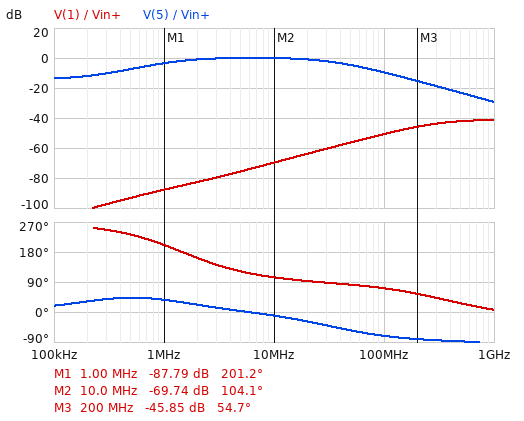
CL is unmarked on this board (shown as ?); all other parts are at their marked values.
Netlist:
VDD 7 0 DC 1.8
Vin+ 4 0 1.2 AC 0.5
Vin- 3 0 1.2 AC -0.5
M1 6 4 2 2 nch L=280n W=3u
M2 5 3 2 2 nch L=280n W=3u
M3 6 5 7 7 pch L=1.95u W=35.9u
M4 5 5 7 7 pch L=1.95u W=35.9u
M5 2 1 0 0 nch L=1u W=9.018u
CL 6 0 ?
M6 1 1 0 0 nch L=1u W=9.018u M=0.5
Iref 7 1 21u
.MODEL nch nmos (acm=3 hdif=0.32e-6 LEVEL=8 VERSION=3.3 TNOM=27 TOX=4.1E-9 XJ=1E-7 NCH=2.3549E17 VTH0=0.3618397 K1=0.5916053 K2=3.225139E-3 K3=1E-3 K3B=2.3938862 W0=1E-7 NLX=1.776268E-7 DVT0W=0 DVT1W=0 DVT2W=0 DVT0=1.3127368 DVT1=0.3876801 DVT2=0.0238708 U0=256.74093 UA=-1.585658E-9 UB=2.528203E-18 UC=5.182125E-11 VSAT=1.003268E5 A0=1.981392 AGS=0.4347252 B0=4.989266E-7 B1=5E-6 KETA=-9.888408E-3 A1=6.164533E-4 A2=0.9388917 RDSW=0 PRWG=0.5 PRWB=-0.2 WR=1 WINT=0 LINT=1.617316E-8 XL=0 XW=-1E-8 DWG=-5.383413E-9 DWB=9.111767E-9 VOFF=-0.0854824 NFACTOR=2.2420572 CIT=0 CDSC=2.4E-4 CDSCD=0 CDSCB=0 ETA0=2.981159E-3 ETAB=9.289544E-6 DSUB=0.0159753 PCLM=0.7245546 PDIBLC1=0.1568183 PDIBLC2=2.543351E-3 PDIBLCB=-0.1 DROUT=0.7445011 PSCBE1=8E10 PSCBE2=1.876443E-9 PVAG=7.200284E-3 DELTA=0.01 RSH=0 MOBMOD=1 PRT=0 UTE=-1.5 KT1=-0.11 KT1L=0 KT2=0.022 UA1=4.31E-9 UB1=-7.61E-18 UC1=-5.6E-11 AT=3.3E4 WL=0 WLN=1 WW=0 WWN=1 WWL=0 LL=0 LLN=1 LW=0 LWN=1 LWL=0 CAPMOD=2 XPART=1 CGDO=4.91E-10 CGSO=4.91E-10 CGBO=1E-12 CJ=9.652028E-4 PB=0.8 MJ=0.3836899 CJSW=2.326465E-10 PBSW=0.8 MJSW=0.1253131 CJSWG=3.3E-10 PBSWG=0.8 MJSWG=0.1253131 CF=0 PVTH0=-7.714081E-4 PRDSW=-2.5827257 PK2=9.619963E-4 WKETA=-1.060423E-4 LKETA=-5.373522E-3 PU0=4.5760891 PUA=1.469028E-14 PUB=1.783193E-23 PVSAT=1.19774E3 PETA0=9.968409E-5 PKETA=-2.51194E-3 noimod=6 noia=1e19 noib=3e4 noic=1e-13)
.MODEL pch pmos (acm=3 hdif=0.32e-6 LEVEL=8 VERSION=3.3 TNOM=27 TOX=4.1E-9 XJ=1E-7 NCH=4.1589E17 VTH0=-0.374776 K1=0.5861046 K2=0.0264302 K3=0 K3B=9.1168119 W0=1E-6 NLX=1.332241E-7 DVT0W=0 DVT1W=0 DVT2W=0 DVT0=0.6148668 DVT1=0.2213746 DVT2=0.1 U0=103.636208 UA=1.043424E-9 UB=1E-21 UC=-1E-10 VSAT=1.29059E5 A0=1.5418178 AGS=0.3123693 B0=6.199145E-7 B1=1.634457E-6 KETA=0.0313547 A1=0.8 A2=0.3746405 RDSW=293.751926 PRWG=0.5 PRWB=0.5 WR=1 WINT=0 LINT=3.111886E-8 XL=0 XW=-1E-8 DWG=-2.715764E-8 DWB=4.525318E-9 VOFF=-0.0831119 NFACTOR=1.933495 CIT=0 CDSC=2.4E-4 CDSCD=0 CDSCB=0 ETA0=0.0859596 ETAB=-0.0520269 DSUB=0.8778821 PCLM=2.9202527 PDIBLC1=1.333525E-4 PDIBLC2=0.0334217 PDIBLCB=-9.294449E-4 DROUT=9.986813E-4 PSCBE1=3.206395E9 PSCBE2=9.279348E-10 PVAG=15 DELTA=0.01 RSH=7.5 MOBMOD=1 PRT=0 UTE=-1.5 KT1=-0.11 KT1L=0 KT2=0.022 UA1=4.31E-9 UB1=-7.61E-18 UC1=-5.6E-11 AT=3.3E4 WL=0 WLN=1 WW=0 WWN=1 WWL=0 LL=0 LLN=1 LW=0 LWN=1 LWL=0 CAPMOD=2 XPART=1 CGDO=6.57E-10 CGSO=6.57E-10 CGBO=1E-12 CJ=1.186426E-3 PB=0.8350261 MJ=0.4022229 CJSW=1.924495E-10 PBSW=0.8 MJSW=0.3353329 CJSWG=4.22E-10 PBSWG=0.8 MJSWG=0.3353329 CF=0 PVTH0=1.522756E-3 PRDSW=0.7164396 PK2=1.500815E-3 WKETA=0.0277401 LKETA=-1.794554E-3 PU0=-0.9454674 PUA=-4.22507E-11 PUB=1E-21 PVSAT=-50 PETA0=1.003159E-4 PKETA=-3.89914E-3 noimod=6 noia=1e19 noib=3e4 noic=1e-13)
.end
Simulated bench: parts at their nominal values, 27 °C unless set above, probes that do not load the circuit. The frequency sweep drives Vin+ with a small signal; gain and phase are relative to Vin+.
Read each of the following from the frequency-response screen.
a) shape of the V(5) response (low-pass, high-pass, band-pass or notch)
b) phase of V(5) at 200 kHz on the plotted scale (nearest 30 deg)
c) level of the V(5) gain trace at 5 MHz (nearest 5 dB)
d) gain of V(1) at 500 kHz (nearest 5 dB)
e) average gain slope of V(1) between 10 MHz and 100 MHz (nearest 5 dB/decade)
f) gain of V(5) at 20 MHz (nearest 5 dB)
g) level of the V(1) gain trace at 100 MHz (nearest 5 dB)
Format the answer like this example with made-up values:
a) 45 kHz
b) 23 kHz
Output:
a) band-pass
b) 30 deg
c) 0 dB
d) -95 dB
e) 20 dB/decade
f) 0 dB
g) -50 dB
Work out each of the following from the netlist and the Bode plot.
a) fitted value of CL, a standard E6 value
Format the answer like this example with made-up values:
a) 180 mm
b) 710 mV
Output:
a) 680 fF
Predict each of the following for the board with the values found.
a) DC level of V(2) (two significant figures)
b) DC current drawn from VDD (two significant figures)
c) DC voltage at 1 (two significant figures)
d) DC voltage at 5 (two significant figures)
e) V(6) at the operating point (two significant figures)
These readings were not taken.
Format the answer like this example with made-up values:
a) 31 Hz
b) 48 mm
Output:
a) 610 mV
b) 63 µA
c) 610 mV
d) 1.2 V
e) 1.2 V
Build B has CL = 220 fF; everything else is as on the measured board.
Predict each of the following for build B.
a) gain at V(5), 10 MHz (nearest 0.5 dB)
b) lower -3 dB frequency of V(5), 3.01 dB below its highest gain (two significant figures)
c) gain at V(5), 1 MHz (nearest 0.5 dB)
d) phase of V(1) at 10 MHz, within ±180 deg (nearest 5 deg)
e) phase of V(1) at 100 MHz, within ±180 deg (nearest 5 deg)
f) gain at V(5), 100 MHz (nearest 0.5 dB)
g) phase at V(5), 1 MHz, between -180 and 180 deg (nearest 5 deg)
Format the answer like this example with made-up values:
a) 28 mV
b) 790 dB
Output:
a) -1.0 dB
b) 2.6 MHz
c) -9.5 dB
d) 125 deg
e) 75 deg
f) -10.0 dB
g) 40 deg
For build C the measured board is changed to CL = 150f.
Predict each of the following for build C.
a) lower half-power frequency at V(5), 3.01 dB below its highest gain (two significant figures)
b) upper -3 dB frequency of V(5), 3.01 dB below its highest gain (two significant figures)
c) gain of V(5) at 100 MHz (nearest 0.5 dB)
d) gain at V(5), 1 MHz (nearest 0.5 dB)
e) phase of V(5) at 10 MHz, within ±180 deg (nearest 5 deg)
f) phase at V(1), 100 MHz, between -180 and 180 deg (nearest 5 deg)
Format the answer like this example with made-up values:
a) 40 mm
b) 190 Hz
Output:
a) 3.2 MHz
b) 42 MHz
c) -10.5 dB
d) -11.0 dB
e) 0 deg
f) 75 deg
